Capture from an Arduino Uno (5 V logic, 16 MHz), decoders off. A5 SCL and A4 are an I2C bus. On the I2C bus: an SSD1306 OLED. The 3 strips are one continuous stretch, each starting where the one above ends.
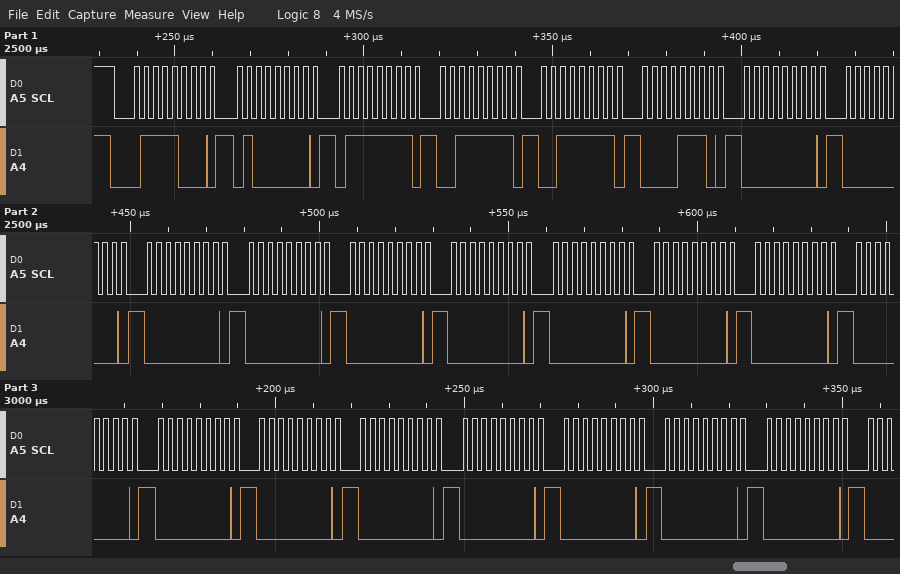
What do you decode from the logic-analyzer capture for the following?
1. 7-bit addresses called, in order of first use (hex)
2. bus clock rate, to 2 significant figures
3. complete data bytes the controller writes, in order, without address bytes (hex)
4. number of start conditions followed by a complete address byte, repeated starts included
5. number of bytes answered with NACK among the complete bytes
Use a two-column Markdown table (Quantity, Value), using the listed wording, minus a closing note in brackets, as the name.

| Quantity | Value |
|---|---|
| 7-bit addresses called, in order of first use | 0x3C |
| bus clock rate, to 2 significant figures | 400 kHz |
| complete data bytes the controller writes, in order, without address bytes | 40 7F 3F 3F 0E 00 00 00 00 00 00 00 00 00 00 00 00 00 00 00 00 00 |
| number of start conditions followed by a complete address byte, repeated starts included | 1 |
| number of bytes answered with NACK among the complete bytes | 0 |
